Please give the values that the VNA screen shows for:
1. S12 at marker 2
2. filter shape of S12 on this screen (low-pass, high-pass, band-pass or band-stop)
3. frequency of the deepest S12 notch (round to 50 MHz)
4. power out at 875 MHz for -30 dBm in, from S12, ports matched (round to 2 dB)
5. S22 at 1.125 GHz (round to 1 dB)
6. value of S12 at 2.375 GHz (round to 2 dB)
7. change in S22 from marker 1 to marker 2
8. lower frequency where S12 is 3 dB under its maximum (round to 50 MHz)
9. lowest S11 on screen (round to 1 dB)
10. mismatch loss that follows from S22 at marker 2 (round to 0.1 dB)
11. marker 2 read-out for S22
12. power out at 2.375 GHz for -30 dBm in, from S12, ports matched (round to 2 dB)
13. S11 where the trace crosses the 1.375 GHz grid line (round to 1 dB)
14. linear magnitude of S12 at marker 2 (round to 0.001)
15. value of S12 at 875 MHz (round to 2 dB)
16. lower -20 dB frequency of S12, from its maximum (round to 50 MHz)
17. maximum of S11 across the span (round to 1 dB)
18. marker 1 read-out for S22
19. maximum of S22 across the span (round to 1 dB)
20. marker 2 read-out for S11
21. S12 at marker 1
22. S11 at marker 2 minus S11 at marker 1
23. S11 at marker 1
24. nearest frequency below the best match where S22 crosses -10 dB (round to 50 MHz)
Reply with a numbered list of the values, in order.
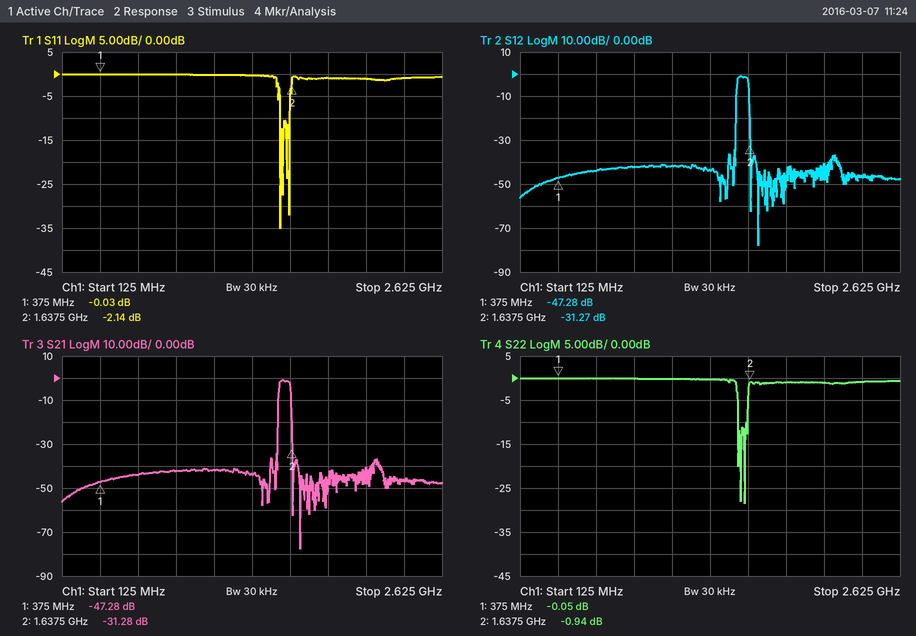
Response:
1. -31.27 dB
2. band-pass
3. 1.70 GHz
4. -72 dBm
5. 0 dB
6. -46 dB
7. -0.89 dB
8. 1.55 GHz
9. -35 dB
10. 7.1 dB
11. -0.94 dB
12. -76 dBm
13. 0 dB
14. 0.027
15. -42 dB
16. 1.55 GHz
17. 0 dB
18. -0.05 dB
19. 0 dB
20. -2.14 dB
21. -47.28 dB
22. -2.11 dB
23. -0.03 dB
24. 1.55 GHz
